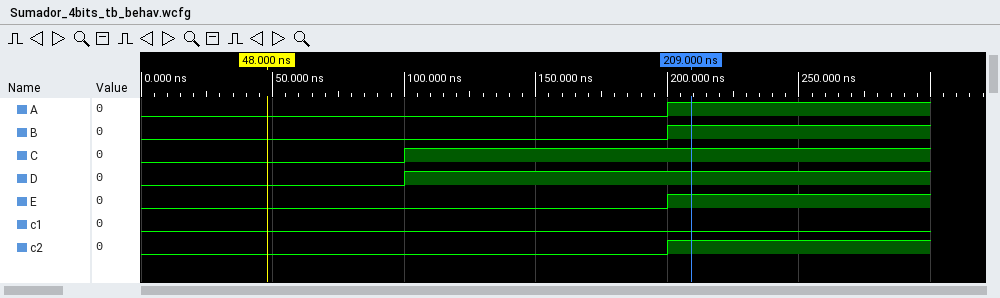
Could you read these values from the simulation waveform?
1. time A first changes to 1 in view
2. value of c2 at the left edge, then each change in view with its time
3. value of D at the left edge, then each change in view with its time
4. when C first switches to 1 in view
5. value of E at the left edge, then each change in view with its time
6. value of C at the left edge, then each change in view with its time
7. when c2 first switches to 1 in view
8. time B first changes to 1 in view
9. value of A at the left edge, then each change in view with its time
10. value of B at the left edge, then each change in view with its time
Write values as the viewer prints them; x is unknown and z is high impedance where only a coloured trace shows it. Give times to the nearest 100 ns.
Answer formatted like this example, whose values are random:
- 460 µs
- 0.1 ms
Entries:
- 200 ns
- 0, 1 at 200 ns
- 0, 1 at 100 ns
- 100 ns
- 0, 1 at 200 ns
- 0, 1 at 100 ns
- 200 ns
- 200 ns
- 0, 1 at 200 ns
- 0, 1 at 200 ns
